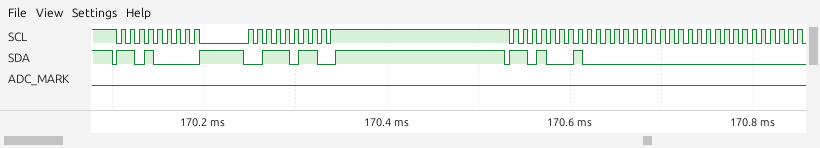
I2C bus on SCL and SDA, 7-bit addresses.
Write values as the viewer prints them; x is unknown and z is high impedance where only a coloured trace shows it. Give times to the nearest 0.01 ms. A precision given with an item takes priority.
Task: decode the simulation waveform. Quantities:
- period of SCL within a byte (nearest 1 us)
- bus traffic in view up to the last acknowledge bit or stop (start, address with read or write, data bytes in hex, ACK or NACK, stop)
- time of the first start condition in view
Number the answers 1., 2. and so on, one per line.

1. 10 us
2. start, address 68 write ACK, 3B ACK, stop, start, address 68 read ACK, 00 ACK, 00 ACK
3. 170.1 ms
